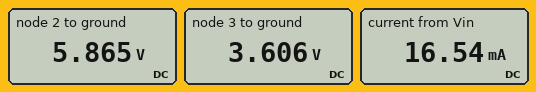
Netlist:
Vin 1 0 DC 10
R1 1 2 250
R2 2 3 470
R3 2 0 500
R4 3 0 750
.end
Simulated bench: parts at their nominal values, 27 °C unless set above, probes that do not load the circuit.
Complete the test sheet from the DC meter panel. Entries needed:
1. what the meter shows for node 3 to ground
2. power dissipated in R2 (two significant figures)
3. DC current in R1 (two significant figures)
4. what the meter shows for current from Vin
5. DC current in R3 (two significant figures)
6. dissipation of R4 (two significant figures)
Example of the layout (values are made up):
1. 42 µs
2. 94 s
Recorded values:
1. 3.606 V
2. 11 mW
3. 17 mA
4. 16.54 mA
5. 12 mA
6. 17 mW
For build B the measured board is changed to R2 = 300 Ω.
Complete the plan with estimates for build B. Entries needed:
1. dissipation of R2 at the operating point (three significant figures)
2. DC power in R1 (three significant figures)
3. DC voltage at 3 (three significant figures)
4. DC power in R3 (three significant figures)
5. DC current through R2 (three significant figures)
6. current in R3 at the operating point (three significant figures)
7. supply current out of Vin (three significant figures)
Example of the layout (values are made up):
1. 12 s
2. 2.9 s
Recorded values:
1. 9.01 mW
2. 72.1 mW
3. 4.11 V
4. 66.2 mW
5. 5.48 mA
6. 11.5 mA
7. 17.0 mA
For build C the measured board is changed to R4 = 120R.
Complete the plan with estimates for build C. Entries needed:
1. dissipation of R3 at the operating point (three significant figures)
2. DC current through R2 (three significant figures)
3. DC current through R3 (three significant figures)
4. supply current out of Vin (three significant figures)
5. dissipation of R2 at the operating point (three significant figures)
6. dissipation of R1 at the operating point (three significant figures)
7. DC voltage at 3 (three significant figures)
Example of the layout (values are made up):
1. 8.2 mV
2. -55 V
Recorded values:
1. 54.0 mW
2. 8.81 mA
3. 10.4 mA
4. 19.2 mA
5. 36.5 mW
6. 92.2 mW
7. 1.06 V
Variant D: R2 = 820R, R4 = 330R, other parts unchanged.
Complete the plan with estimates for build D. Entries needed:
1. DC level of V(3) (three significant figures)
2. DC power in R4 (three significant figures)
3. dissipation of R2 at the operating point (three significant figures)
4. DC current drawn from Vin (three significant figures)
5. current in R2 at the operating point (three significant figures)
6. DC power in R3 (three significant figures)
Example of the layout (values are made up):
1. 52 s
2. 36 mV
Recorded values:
1. 1.67 V
2. 8.46 mW
3. 21.0 mW
4. 16.7 mA
5. 5.06 mA
6. 67.8 mW
